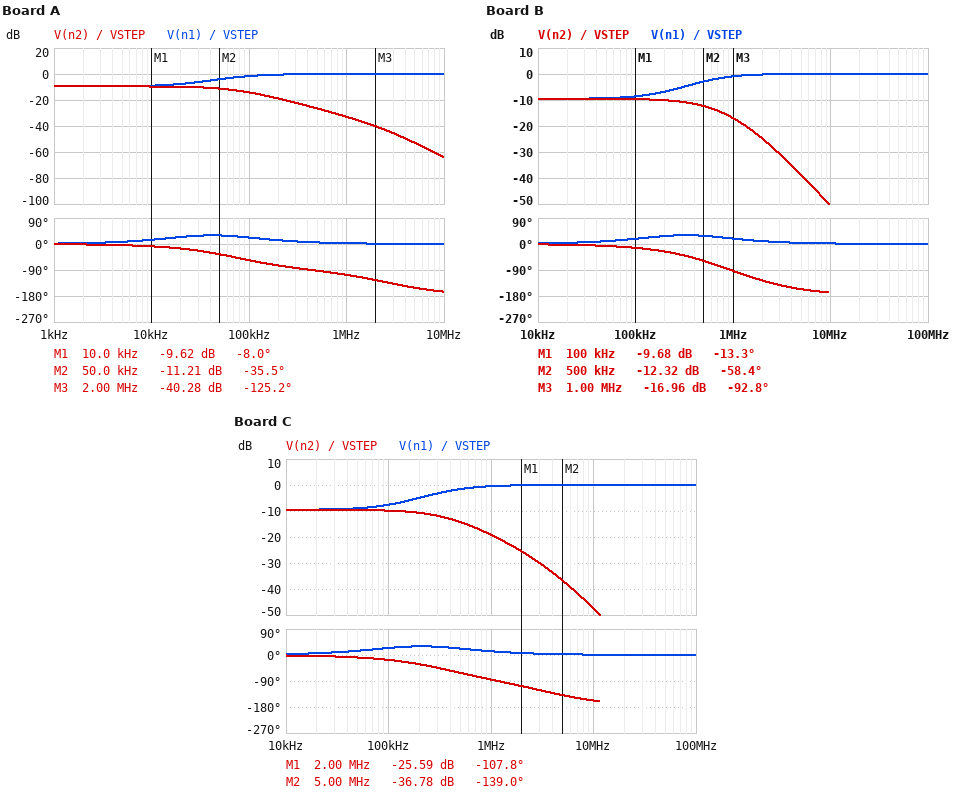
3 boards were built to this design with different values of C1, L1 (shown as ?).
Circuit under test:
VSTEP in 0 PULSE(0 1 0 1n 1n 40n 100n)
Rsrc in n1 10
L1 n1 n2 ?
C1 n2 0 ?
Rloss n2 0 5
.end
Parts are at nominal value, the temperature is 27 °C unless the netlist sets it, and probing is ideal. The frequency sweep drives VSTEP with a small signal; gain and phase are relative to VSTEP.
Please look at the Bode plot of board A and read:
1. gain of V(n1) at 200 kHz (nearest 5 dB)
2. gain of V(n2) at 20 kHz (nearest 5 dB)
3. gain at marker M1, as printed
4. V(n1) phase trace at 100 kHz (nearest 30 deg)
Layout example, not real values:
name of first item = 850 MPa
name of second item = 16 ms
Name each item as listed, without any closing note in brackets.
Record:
gain of V(n1) at 200 kHz = 0 dB
gain of V(n2) at 20 kHz = -10 dB
gain at marker M1, as printed = -9.62 dB
V(n1) phase trace at 100 kHz = 30 deg
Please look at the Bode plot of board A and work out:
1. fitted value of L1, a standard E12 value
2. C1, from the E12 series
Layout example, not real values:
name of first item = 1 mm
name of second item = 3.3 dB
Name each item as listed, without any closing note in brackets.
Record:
fitted value of L1, a standard E12 value = 33 µH
C1, from the E12 series = 12 nF
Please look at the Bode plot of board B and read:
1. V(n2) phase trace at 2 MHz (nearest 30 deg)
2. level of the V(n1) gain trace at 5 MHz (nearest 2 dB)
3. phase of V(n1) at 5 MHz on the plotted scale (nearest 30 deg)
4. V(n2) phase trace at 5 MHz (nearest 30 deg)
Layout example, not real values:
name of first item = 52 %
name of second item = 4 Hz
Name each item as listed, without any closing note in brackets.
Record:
V(n2) phase trace at 2 MHz = -120 deg
level of the V(n1) gain trace at 5 MHz = 0 dB
phase of V(n1) at 5 MHz on the plotted scale = 0 deg
V(n2) phase trace at 5 MHz = -150 deg
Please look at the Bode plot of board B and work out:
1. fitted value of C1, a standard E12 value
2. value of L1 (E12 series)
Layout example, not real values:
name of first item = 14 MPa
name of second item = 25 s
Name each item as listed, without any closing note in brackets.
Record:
fitted value of C1, a standard E12 value = 18 nF
value of L1 = 4.7 µH
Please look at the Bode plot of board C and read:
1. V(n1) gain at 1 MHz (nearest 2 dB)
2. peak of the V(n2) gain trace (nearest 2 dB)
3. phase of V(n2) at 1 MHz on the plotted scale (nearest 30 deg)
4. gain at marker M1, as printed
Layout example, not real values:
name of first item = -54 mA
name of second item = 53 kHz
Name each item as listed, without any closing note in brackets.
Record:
V(n1) gain at 1 MHz = 0 dB
peak of the V(n2) gain trace = -10 dB
phase of V(n2) at 1 MHz on the plotted scale = -90 deg
gain at marker M1, as printed = -25.59 dB
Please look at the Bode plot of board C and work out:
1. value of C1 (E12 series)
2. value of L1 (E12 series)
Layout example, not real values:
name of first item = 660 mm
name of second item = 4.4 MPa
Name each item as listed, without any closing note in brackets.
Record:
value of C1 = 8.2 nF
value of L1 = 6.8 µH
